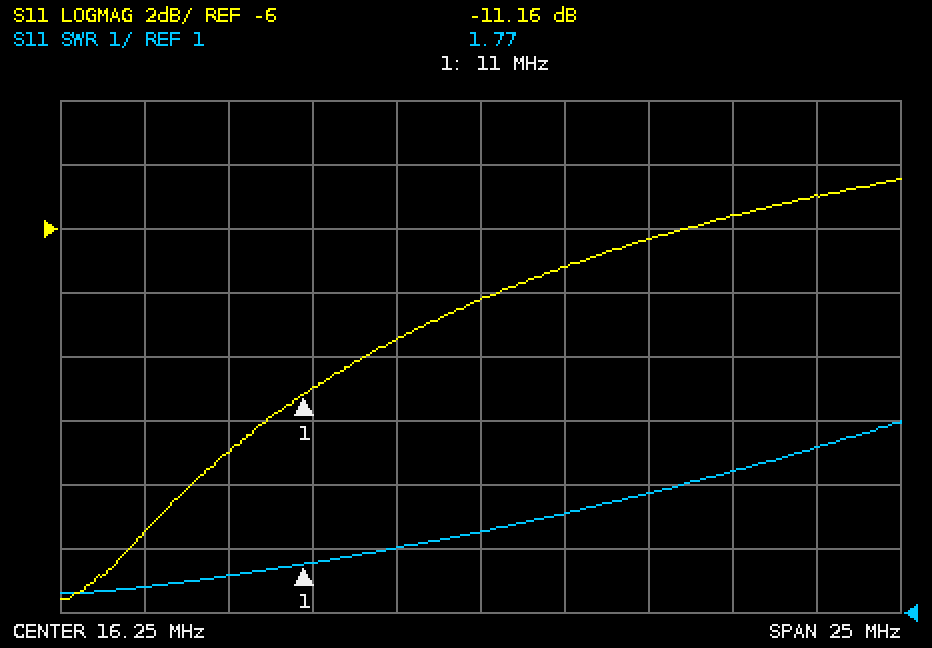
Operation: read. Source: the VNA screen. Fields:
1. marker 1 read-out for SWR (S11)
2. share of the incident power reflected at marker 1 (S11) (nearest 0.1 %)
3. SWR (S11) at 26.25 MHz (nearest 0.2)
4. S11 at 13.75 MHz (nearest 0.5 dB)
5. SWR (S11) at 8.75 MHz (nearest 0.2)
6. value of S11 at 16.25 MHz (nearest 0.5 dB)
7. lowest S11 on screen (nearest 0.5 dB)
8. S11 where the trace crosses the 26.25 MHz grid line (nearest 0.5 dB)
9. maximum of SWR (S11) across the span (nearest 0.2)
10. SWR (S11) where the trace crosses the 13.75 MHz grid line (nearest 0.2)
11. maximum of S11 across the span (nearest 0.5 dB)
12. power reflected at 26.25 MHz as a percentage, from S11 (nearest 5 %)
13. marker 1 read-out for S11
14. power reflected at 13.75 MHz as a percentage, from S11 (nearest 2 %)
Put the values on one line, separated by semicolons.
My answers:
1.77; 7.7 %; 3.6; -9.5 dB; 1.6; -8.0 dB; -17.5 dB; -5.0 dB; 4.0; 2.0; -4.5 dB; 30 %; -11.16 dB; 12 %
